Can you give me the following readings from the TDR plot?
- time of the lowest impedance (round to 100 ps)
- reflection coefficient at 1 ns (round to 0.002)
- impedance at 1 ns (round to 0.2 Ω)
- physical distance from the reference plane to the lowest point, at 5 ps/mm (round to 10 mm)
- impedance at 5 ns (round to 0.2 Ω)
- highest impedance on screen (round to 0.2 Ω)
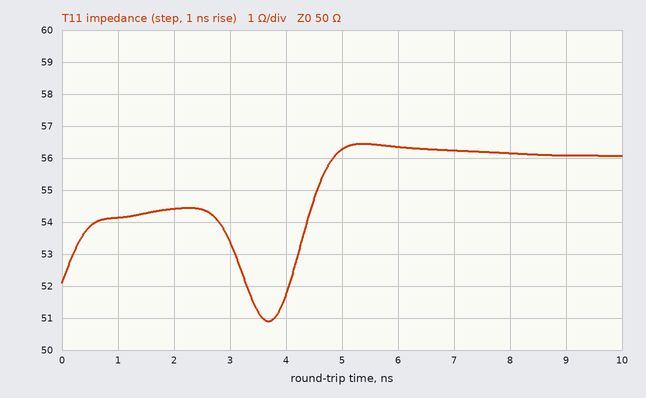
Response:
3.7 ns
+0.040
54.2 Ω
370 mm
56.2 Ω
56.4 Ω
